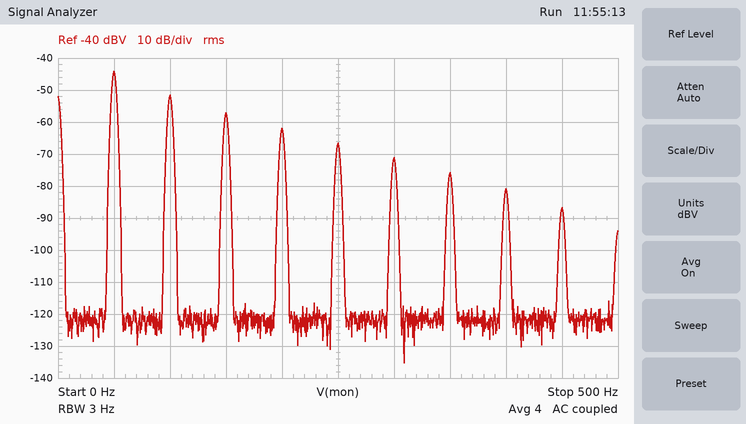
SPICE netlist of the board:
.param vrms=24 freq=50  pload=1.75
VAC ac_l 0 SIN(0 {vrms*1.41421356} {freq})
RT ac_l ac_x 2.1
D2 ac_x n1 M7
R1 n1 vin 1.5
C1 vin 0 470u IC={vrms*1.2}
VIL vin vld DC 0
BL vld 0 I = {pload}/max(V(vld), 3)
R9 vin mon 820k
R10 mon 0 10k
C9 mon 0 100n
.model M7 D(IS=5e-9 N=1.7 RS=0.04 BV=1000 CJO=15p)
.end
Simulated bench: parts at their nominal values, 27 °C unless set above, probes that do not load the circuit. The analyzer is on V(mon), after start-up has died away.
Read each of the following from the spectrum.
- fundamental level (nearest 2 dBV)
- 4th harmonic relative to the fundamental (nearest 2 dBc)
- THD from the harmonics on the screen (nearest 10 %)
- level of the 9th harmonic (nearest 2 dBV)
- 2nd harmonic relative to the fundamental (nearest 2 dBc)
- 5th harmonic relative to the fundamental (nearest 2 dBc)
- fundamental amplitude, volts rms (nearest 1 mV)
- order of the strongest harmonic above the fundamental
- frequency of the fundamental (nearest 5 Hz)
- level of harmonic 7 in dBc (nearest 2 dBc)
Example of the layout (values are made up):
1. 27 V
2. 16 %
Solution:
1. -44 dBV
2. -18 dBc
3. 50 %
4. -86 dBV
5. -8 dBc
6. -22 dBc
7. 6 mV
8. 2
9. 50 Hz
10. -32 dBc
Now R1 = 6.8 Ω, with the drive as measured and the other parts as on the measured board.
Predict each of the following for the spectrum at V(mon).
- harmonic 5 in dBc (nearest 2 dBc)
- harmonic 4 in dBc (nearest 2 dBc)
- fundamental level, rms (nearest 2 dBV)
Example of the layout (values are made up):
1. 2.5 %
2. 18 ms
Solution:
1. -26 dBc
2. -20 dBc
3. -44 dBV
